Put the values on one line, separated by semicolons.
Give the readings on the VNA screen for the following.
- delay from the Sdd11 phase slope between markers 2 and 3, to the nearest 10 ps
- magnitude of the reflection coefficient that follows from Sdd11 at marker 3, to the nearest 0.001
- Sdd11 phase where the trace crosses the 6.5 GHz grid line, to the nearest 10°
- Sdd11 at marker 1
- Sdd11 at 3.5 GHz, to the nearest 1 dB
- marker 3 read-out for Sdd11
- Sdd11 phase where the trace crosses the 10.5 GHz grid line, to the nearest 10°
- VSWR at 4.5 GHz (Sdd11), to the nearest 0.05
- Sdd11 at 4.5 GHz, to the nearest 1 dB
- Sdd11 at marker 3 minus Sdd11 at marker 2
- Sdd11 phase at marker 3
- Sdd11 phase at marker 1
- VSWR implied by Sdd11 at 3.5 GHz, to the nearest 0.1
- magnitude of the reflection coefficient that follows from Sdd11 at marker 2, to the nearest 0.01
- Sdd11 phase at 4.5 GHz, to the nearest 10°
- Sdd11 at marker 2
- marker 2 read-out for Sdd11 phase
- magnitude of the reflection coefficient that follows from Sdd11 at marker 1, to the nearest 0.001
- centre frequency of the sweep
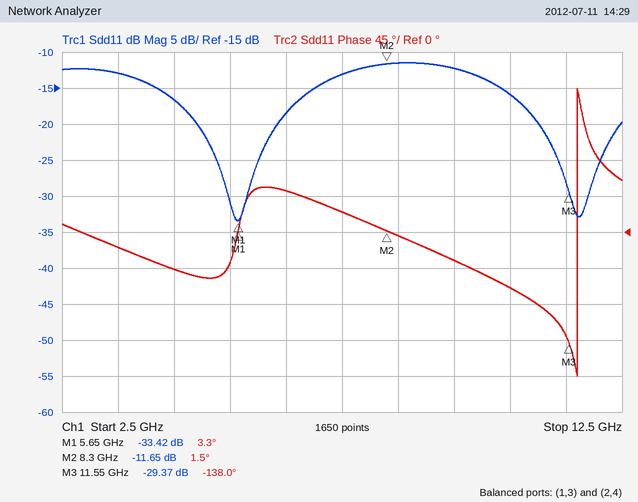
120 ps; 0.034; 50°; -33.42 dB; -13 dB; -29.37 dB; -70°; 1.35; -17 dB; -17.72 dB; -138.0°; 3.3°; 1.6; 0.26; -50°; -11.65 dB; 1.5°; 0.021; 7.5 GHz
